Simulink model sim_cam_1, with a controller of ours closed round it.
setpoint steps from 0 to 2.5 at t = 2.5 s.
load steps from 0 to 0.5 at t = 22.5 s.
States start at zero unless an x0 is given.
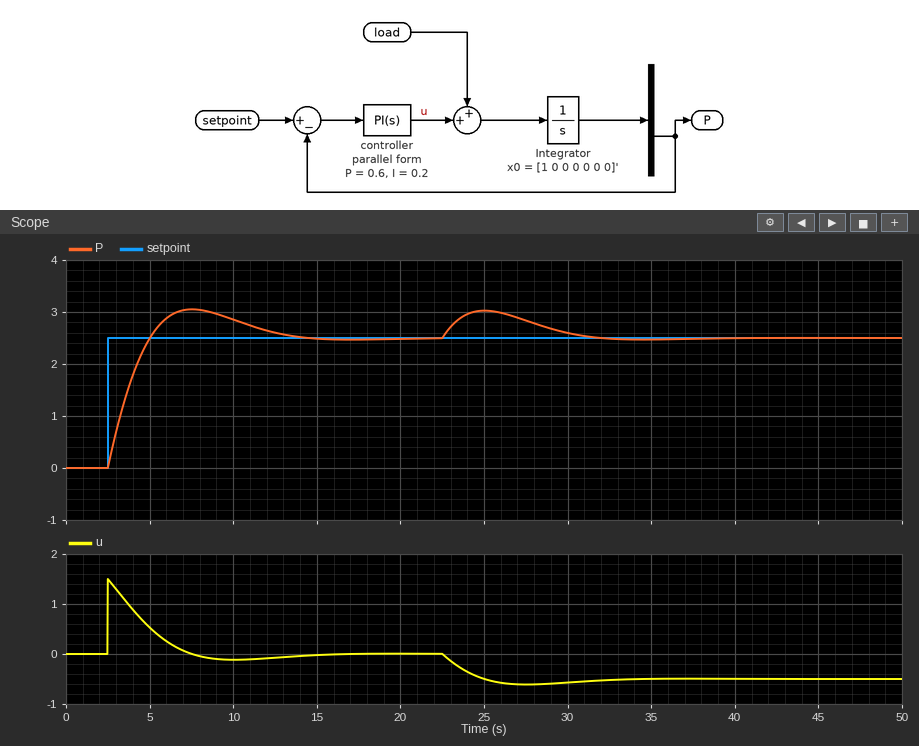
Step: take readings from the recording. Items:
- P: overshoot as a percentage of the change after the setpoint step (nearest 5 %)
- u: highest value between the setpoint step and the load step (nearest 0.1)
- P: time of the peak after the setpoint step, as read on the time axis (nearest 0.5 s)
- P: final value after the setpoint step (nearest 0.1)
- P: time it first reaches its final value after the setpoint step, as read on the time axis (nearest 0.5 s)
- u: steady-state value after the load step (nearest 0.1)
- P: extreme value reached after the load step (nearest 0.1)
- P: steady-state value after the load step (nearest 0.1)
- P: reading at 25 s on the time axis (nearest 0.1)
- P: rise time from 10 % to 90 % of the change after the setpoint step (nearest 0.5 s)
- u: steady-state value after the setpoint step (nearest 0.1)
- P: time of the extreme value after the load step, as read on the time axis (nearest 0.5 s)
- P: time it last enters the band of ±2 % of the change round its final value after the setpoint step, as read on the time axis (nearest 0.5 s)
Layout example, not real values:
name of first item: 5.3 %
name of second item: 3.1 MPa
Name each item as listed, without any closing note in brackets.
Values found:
P: overshoot as a percentage of the change after the setpoint step: 20 %
u: highest value between the setpoint step and the load step: 1.5
P: time of the peak after the setpoint step, as read on the time axis: 7.5 s
P: final value after the setpoint step: 2.5
P: time it first reaches its final value after the setpoint step, as read on the time axis: 5.0 s
u: steady-state value after the load step: -0.5
P: extreme value reached after the load step: 3.0
P: steady-state value after the load step: 2.5
P: reading at 25 s on the time axis: 3.0
P: rise time from 10 % to 90 % of the change after the setpoint step: 2.0 s
u: steady-state value after the setpoint step: 0.0
P: time of the extreme value after the load step, as read on the time axis: 25.0 s
P: time it last enters the band of ±2 % of the change round its final value after the setpoint step, as read on the time axis: 13.5 s
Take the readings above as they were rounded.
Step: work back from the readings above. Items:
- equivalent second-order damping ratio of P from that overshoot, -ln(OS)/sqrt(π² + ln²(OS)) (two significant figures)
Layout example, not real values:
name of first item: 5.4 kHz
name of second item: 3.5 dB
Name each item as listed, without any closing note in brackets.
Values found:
equivalent second-order damping ratio of P from that overshoot, -ln(OS)/sqrt(π² + ln²(OS)): 0.46
